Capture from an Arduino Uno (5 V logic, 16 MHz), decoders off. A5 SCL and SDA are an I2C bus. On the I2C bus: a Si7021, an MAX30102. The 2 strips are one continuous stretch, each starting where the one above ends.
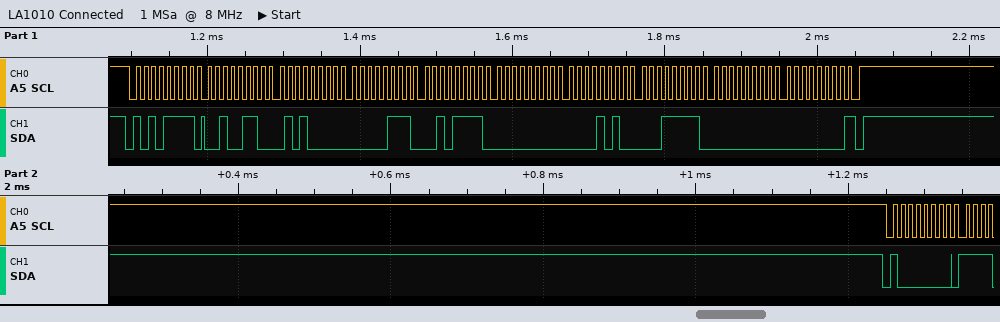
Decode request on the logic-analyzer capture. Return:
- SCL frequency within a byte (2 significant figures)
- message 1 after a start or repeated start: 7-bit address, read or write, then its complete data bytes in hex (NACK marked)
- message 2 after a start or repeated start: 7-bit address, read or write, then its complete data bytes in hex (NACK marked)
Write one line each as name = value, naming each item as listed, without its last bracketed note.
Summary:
SCL frequency within a byte = 100 kHz
message 1 after a start or repeated start: 7-bit address, read or write, then its complete data bytes in hex = 0x57 read: 26 50 07 2F 00 0A 1F 00 00 NACK
message 2 after a start or repeated start: 7-bit address, read or write, then its complete data bytes in hex = 0x40 write
